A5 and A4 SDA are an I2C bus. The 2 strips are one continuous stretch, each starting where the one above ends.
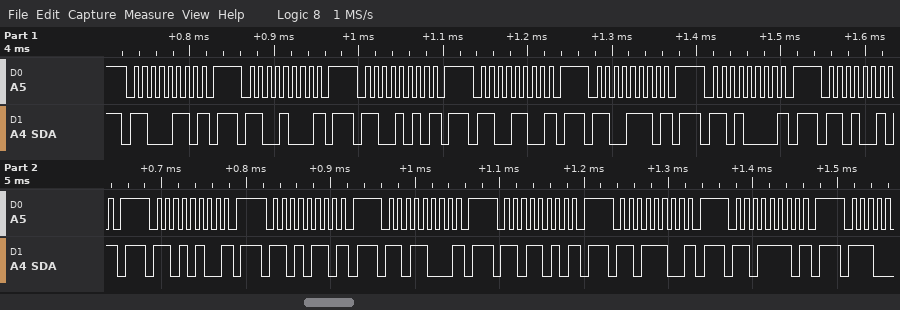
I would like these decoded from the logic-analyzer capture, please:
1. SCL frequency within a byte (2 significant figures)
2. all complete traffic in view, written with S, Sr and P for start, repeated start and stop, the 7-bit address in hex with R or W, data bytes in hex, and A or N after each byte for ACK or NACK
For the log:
100 kHz
S 63W N P S 64W N P S 65W N P S 66W N P S 67W N P S 68W N P S 69W N P S 6AW N P S 6BW N P S 6CW N P S 6DW N P S 6EW N P S 6FW N P
